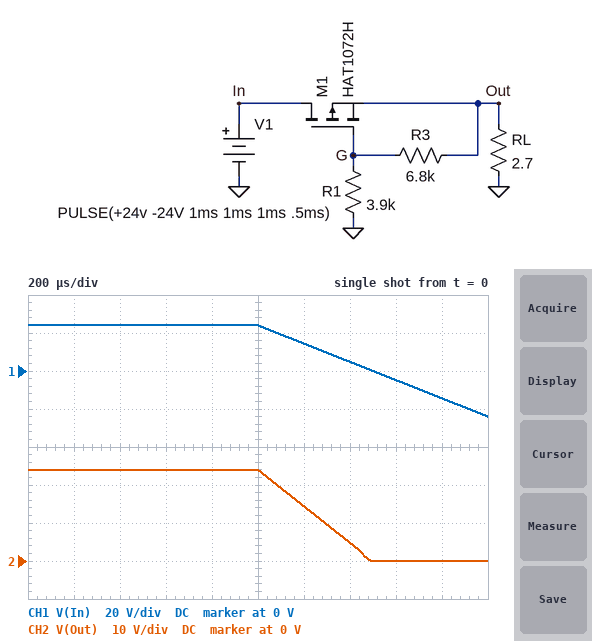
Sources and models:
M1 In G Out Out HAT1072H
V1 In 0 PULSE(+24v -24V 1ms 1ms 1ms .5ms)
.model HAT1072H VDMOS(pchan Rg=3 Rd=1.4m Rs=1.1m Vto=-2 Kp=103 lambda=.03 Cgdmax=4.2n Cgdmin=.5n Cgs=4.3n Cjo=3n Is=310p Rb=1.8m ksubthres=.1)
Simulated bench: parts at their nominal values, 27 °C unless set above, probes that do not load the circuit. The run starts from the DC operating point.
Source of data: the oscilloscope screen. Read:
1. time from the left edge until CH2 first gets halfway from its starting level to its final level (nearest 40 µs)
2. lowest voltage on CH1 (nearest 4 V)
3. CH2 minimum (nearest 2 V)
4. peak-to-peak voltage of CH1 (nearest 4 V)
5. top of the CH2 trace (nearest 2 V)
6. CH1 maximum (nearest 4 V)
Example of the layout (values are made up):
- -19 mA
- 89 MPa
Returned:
- 1.24 ms
- -24 V
- 0 V
- 48 V
- 24 V
- 24 V
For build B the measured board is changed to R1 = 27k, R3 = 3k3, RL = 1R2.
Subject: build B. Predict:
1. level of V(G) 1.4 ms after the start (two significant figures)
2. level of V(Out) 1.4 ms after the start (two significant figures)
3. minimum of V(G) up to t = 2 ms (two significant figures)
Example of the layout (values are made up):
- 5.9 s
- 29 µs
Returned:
- 3.6 V
- 4.2 V
- -320 mV
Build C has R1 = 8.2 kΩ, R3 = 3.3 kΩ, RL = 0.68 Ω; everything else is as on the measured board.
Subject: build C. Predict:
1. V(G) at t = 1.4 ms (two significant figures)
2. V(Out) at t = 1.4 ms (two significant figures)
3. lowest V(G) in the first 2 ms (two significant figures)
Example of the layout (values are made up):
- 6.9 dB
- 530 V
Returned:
- 2.7 V
- 4.2 V
- -330 mV
